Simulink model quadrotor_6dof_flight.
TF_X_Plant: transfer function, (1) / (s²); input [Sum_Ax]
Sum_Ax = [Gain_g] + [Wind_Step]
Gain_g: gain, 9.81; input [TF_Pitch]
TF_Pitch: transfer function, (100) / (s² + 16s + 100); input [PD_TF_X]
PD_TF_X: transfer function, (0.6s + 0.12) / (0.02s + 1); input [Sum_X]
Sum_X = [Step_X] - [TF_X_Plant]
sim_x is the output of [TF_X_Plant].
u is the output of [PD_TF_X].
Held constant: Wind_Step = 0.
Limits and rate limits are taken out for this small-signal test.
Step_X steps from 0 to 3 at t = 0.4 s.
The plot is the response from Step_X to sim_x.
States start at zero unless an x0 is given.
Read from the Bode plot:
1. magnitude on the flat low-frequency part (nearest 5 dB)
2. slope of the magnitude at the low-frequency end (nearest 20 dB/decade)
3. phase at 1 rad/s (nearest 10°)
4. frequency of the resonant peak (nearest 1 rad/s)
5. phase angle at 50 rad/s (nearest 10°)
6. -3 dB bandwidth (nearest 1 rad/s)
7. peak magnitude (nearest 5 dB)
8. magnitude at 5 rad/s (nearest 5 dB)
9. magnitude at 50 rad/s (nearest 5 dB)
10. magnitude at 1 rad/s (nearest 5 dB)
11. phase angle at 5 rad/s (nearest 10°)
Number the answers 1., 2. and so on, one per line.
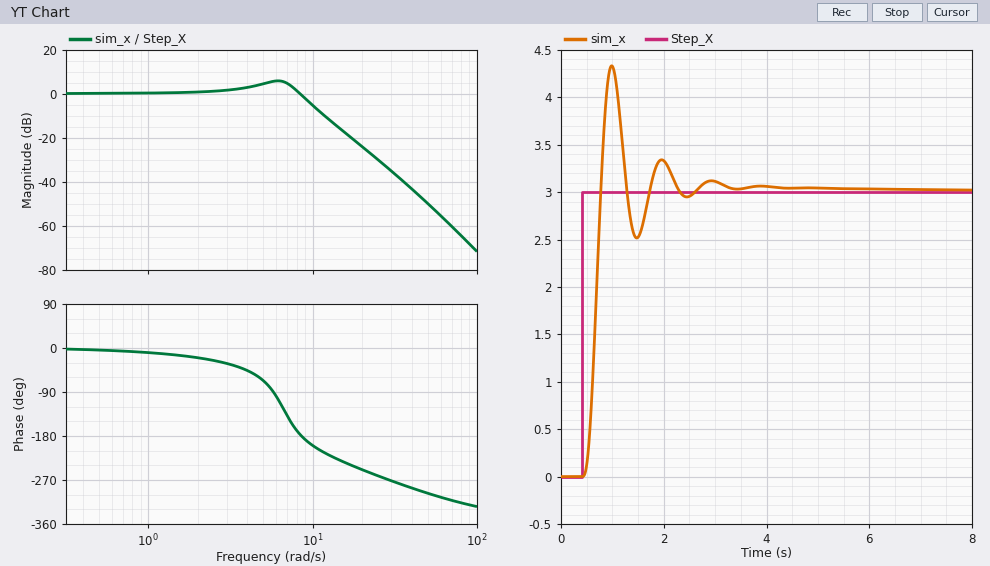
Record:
1. 0 dB
2. 0 dB/decade
3. -10°
4. 6 rad/s
5. -300°
6. 9 rad/s
7. 5 dB
8. 5 dB
9. -50 dB
10. 0 dB
11. -70°
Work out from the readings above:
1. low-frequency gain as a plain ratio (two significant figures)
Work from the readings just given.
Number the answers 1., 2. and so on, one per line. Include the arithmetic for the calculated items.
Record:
1. 10^(0 / 20) = 1.0
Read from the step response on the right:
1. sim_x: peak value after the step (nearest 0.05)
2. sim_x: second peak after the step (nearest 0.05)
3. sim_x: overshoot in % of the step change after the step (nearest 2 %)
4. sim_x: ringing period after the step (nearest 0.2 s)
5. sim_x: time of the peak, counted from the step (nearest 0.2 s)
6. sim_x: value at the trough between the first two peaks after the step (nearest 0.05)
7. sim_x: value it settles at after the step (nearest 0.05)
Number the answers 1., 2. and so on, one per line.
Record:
1. 4.35
2. 3.35
3. 44 %
4. 1.0 s
5. 0.6 s
6. 2.50
7. 3.00
